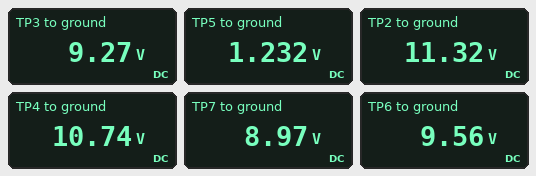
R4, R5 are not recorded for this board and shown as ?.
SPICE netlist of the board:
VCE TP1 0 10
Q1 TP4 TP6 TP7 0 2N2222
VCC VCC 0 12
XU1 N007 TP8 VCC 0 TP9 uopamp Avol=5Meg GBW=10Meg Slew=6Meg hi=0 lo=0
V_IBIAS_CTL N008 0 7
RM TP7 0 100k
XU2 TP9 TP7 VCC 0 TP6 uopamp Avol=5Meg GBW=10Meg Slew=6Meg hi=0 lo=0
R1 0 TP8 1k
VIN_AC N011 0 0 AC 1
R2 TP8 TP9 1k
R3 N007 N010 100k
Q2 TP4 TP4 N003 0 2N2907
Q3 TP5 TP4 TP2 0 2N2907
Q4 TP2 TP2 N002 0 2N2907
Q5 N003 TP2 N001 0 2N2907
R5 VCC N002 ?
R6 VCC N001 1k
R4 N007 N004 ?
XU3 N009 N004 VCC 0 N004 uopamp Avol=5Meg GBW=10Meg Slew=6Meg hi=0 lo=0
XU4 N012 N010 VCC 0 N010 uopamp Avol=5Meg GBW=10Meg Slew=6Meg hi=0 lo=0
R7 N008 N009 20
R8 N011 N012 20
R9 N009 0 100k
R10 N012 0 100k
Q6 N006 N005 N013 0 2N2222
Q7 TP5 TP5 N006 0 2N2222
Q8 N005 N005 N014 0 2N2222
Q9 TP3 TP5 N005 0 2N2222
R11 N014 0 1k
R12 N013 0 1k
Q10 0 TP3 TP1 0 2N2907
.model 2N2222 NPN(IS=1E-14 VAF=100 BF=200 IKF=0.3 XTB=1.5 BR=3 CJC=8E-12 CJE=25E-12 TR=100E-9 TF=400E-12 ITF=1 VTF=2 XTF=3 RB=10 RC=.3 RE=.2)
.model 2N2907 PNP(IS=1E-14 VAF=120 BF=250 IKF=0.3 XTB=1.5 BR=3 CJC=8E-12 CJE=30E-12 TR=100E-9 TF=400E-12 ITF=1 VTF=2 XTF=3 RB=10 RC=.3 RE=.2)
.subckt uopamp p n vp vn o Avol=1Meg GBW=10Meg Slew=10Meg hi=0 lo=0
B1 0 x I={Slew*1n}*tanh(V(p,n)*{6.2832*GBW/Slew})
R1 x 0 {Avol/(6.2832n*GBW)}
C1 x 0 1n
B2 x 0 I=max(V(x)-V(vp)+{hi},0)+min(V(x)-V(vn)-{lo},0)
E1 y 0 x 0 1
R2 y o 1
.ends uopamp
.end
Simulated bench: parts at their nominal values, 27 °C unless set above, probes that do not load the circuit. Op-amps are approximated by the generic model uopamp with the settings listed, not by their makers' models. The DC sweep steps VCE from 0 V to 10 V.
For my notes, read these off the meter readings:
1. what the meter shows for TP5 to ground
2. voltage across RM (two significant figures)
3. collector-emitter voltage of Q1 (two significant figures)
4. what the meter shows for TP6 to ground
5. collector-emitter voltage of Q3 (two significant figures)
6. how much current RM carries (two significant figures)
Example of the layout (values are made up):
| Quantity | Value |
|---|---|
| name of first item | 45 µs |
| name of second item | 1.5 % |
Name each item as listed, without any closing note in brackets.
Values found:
| Quantity | Value |
|---|---|
| what the meter shows for TP5 to ground | 1.232 V |
| voltage across RM | 9.0 V |
| collector-emitter voltage of Q1 | 1.8 V |
| what the meter shows for TP6 to ground | 9.56 V |
| collector-emitter voltage of Q3 | -10 V |
| how much current RM carries | 90 µA |
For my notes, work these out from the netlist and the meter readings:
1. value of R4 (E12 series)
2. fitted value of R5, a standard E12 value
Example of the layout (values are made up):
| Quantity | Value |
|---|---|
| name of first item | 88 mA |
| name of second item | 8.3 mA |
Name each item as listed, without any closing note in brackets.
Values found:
| Quantity | Value |
|---|---|
| value of R4 | 56 kΩ |
| fitted value of R5, a standard E12 value | 1.5 kΩ |
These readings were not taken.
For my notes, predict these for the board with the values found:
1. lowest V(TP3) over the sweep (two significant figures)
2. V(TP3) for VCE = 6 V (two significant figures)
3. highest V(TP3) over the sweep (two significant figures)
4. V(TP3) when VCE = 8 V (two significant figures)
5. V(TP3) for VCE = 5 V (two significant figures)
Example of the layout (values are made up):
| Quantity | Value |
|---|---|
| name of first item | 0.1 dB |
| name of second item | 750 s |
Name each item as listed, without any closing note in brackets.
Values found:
| Quantity | Value |
|---|---|
| lowest V(TP3) over the sweep | 610 mV |
| V(TP3) for VCE = 6 V | 5.3 V |
| highest V(TP3) over the sweep | 9.3 V |
| V(TP3) when VCE = 8 V | 7.3 V |
| V(TP3) for VCE = 5 V | 4.3 V |
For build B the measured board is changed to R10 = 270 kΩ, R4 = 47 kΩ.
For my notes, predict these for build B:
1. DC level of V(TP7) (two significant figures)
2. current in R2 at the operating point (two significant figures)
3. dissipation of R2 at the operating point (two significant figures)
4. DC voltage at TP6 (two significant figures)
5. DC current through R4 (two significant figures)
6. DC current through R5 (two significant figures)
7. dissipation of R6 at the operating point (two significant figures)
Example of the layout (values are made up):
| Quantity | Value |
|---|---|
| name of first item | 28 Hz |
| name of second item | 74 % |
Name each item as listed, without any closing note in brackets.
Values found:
| Quantity | Value |
|---|---|
| DC level of V(TP7) | 9.5 V |
| current in R2 at the operating point | 4.8 mA |
| dissipation of R2 at the operating point | 23 mW |
| DC voltage at TP6 | 10 V |
| DC current through R4 | 48 µA |
| DC current through R5 | 69 µA |
| dissipation of R6 at the operating point | 9.0 µW |
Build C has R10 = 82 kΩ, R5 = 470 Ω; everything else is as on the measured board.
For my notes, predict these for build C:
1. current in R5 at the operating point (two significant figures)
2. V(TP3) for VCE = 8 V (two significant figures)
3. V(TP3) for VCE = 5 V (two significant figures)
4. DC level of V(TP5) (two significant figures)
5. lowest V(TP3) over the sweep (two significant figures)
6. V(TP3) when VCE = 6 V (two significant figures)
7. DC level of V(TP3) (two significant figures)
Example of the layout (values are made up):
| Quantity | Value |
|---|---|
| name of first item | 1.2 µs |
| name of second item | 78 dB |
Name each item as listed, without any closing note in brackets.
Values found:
| Quantity | Value |
|---|---|
| current in R5 at the operating point | 160 µA |
| V(TP3) for VCE = 8 V | 7.2 V |
| V(TP3) for VCE = 5 V | 4.2 V |
| DC level of V(TP5) | 1.4 V |
| lowest V(TP3) over the sweep | 680 mV |
| V(TP3) when VCE = 6 V | 5.2 V |
| DC level of V(TP3) | 9.2 V |
